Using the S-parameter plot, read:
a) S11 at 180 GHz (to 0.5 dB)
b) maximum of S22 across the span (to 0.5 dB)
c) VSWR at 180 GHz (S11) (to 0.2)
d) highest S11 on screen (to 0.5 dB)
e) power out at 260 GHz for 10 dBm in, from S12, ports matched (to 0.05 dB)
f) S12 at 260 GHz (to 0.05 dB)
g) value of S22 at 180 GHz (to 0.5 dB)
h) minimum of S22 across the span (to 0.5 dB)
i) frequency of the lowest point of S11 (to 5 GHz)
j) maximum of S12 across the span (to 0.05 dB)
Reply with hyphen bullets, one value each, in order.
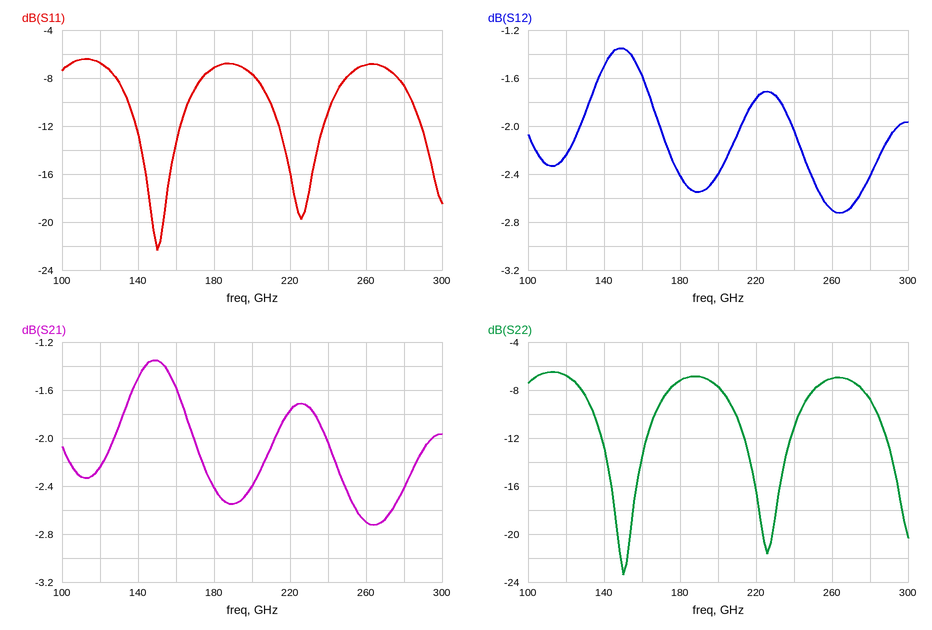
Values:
- -7.0 dB
- -6.5 dB
- 2.6
- -6.5 dB
- 7.30 dBm
- -2.70 dB
- -7.0 dB
- -23.5 dB
- 150 GHz
- -1.35 dB
